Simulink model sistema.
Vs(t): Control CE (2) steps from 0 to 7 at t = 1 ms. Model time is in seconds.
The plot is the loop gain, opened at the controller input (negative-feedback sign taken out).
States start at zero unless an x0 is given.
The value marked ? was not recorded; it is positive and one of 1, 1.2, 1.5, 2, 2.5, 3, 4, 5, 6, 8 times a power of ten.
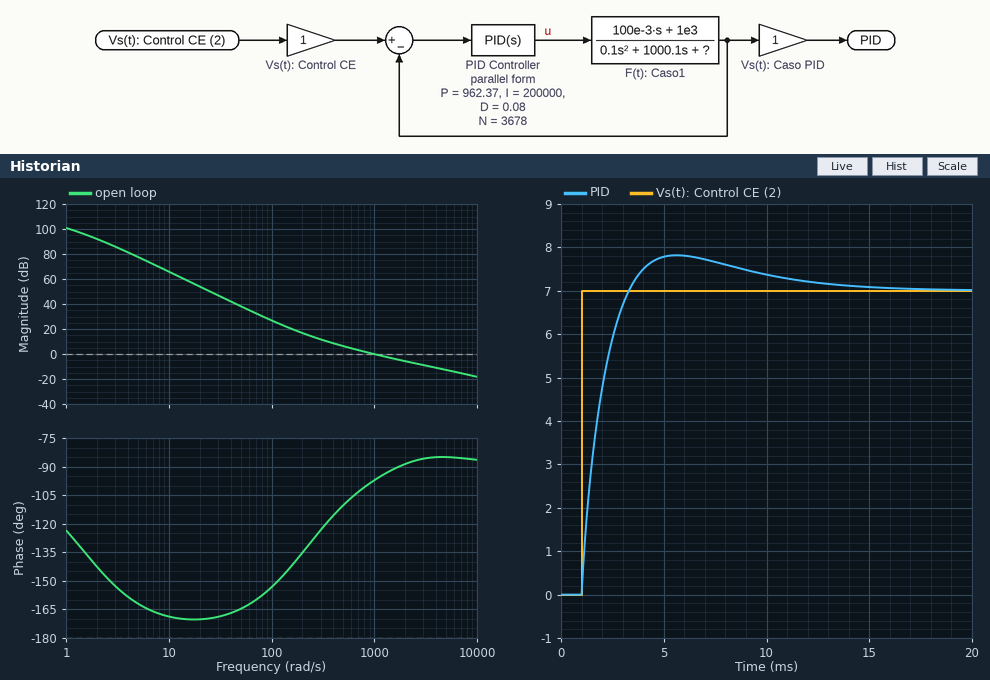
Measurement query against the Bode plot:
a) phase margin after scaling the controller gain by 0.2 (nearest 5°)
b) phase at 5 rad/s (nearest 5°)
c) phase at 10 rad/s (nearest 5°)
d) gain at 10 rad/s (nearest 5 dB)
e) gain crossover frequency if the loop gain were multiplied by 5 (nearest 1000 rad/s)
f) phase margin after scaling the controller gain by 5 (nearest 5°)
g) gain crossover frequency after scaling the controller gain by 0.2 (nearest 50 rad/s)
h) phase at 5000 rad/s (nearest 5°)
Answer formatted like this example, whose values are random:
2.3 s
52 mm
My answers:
50°
-160°
-170°
65 dB
6000 rad/s
95°
250 rad/s
-85°
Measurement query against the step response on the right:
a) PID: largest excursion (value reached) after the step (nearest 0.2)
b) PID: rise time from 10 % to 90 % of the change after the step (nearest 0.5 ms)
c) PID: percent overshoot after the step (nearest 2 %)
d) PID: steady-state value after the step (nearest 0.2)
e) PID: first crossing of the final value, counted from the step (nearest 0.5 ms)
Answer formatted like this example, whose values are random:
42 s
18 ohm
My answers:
7.8
1.5 ms
12 %
7.0
2.5 ms
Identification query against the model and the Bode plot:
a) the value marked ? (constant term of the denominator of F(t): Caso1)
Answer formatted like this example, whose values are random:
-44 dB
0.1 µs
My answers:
1500
